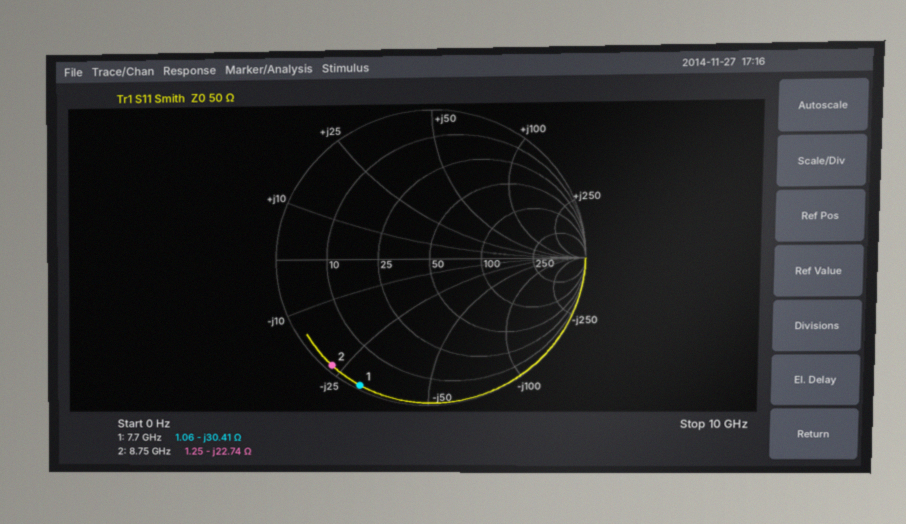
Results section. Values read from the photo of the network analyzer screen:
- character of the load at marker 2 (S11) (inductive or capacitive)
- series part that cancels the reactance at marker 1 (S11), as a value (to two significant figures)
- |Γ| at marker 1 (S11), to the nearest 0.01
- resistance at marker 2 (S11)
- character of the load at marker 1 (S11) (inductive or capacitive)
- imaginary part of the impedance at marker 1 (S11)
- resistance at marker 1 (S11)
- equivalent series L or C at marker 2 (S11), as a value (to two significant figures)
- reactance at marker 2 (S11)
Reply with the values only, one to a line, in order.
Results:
capacitive
630 pH
0.97
1.25 Ω
capacitive
-30.41 Ω
1.06 Ω
800 fF
-22.74 Ω
